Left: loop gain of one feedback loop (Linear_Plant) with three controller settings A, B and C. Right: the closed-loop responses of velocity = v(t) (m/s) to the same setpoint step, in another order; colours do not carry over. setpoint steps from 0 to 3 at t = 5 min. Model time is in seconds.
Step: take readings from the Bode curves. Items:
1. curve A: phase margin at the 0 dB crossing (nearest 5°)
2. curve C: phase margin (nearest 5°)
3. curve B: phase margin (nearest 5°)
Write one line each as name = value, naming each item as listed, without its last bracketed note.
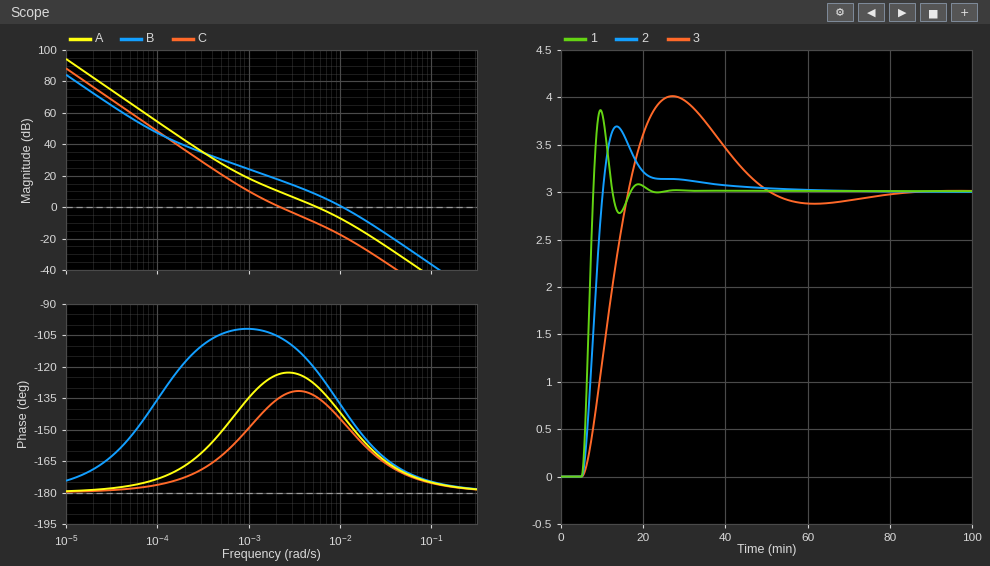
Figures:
curve A: phase margin at the 0 dB crossing = 50°
curve C: phase margin = 45°
curve B: phase margin = 40°
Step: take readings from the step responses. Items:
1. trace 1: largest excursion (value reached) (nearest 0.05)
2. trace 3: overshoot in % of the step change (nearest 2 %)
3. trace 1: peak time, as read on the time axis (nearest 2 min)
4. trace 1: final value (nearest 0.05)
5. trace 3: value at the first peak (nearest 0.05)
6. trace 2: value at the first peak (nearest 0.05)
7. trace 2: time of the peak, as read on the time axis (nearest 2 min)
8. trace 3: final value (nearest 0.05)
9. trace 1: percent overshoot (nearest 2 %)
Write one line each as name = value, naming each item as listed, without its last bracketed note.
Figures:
trace 1: largest excursion (value reached) = 3.85
trace 3: overshoot in % of the step change = 34 %
trace 1: peak time, as read on the time axis = 10 min
trace 1: final value = 3.00
trace 3: value at the first peak = 4.00
trace 2: value at the first peak = 3.70
trace 2: time of the peak, as read on the time axis = 14 min
trace 3: final value = 3.00
trace 1: percent overshoot = 28 %
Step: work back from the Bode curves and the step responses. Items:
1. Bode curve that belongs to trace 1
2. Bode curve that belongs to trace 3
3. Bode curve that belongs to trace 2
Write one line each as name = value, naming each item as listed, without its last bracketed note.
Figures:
Bode curve that belongs to trace 1 = B
Bode curve that belongs to trace 3 = C
Bode curve that belongs to trace 2 = A
